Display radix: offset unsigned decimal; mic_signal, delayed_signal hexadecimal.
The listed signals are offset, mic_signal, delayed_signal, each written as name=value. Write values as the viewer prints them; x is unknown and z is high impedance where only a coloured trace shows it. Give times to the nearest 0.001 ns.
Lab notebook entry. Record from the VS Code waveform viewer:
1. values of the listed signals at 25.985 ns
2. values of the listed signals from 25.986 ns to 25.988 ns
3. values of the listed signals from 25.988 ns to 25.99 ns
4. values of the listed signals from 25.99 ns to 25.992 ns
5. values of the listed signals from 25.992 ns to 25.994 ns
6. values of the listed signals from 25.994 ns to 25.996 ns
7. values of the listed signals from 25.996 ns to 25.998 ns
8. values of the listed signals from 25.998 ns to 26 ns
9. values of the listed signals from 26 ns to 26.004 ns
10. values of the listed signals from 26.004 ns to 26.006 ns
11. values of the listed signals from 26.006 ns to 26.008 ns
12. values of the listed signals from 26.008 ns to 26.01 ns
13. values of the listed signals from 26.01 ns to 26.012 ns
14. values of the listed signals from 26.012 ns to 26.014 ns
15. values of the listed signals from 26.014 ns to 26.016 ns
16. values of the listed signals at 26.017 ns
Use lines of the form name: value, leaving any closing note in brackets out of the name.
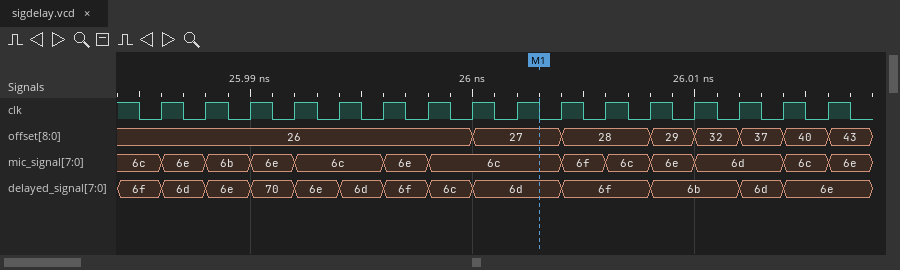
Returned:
values of the listed signals at 25.985 ns: offset=26, mic_signal=6c, delayed_signal=6f
values of the listed signals from 25.986 ns to 25.988 ns: offset=26, mic_signal=6e, delayed_signal=6d
values of the listed signals from 25.988 ns to 25.99 ns: offset=26, mic_signal=6b, delayed_signal=6e
values of the listed signals from 25.99 ns to 25.992 ns: offset=26, mic_signal=6e, delayed_signal=70
values of the listed signals from 25.992 ns to 25.994 ns: offset=26, mic_signal=6c, delayed_signal=6e
values of the listed signals from 25.994 ns to 25.996 ns: offset=26, mic_signal=6c, delayed_signal=6d
values of the listed signals from 25.996 ns to 25.998 ns: offset=26, mic_signal=6e, delayed_signal=6f
values of the listed signals from 25.998 ns to 26 ns: offset=26, mic_signal=6c, delayed_signal=6c
values of the listed signals from 26 ns to 26.004 ns: offset=27, mic_signal=6c, delayed_signal=6d
values of the listed signals from 26.004 ns to 26.006 ns: offset=28, mic_signal=6f, delayed_signal=6f
values of the listed signals from 26.006 ns to 26.008 ns: offset=28, mic_signal=6c, delayed_signal=6f
values of the listed signals from 26.008 ns to 26.01 ns: offset=29, mic_signal=6e, delayed_signal=6b
values of the listed signals from 26.01 ns to 26.012 ns: offset=32, mic_signal=6d, delayed_signal=6b
values of the listed signals from 26.012 ns to 26.014 ns: offset=37, mic_signal=6d, delayed_signal=6d
values of the listed signals from 26.014 ns to 26.016 ns: offset=40, mic_signal=6c, delayed_signal=6e
values of the listed signals at 26.017 ns: offset=43, mic_signal=6e, delayed_signal=6e
